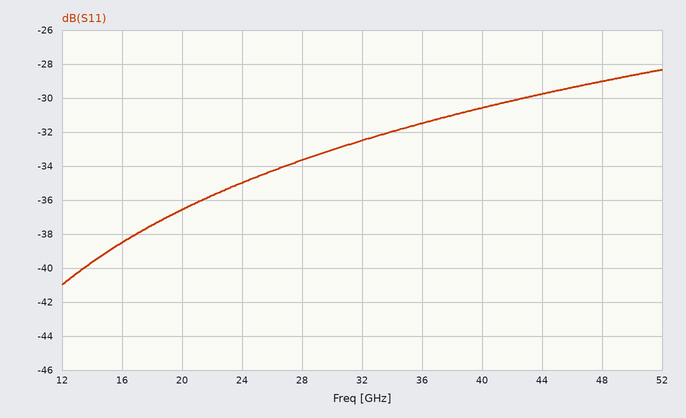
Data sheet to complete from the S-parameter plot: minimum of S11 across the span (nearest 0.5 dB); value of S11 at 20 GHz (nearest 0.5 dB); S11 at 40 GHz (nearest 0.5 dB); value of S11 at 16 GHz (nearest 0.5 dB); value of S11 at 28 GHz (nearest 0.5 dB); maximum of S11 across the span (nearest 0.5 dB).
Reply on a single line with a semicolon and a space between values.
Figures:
-41.0 dB; -36.5 dB; -30.5 dB; -38.5 dB; -33.5 dB; -28.5 dB
